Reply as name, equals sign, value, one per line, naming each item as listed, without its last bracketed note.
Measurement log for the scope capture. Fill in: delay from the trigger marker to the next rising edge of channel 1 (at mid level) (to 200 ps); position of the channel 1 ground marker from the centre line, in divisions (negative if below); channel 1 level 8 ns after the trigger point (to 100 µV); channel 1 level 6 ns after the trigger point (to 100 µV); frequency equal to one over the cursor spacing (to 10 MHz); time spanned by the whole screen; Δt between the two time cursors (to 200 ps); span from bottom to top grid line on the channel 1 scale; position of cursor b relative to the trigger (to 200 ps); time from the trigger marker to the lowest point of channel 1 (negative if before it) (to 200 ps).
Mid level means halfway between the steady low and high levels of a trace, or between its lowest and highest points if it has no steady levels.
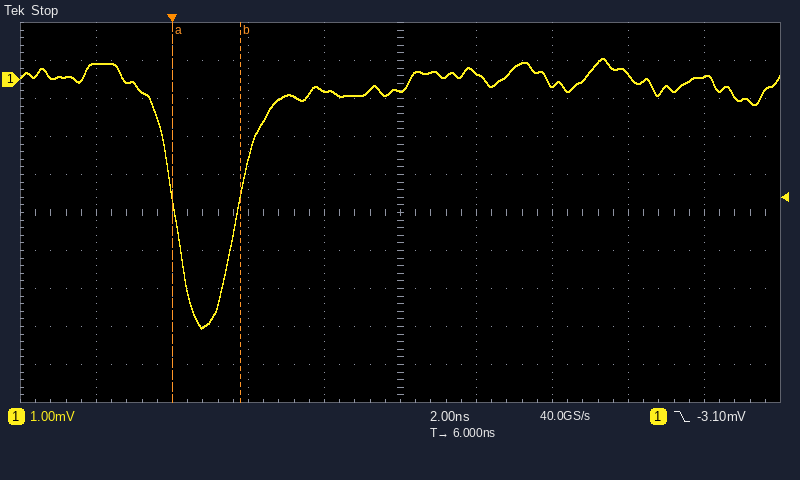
delay from the trigger marker to the next rising edge of channel 1 (at mid level) = 1.8 ns
position of the channel 1 ground marker from the centre line, in divisions = +3.5 div
channel 1 level 8 ns after the trigger point = 200 µV
channel 1 level 6 ns after the trigger point = -300 µV
frequency equal to one over the cursor spacing = 560 MHz
time spanned by the whole screen = 20 ns
Δt between the two time cursors = 1.8 ns
span from bottom to top grid line on the channel 1 scale = 10 mV
position of cursor b relative to the trigger = +1.8 ns
time from the trigger marker to the lowest point of channel 1 (negative if before it) = +800 ps
